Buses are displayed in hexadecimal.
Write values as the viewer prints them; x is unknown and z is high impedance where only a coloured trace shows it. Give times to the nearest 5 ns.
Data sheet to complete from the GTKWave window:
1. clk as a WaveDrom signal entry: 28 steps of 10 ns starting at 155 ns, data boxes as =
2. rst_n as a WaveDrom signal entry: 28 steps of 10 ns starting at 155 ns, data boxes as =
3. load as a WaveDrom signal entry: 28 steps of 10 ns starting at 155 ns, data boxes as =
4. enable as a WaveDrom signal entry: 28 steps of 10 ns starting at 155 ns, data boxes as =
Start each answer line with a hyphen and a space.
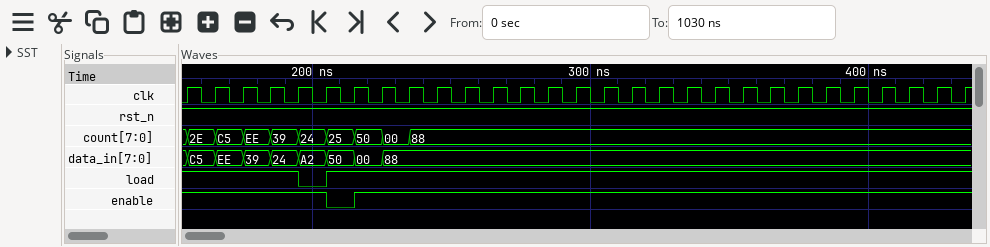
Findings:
- {name: 'clk', wave: 'p...........................'}
- {name: 'rst_n', wave: '1...........................'}
- {name: 'load', wave: '1...01......................'}
- {name: 'enable', wave: '1....01.....................'}
